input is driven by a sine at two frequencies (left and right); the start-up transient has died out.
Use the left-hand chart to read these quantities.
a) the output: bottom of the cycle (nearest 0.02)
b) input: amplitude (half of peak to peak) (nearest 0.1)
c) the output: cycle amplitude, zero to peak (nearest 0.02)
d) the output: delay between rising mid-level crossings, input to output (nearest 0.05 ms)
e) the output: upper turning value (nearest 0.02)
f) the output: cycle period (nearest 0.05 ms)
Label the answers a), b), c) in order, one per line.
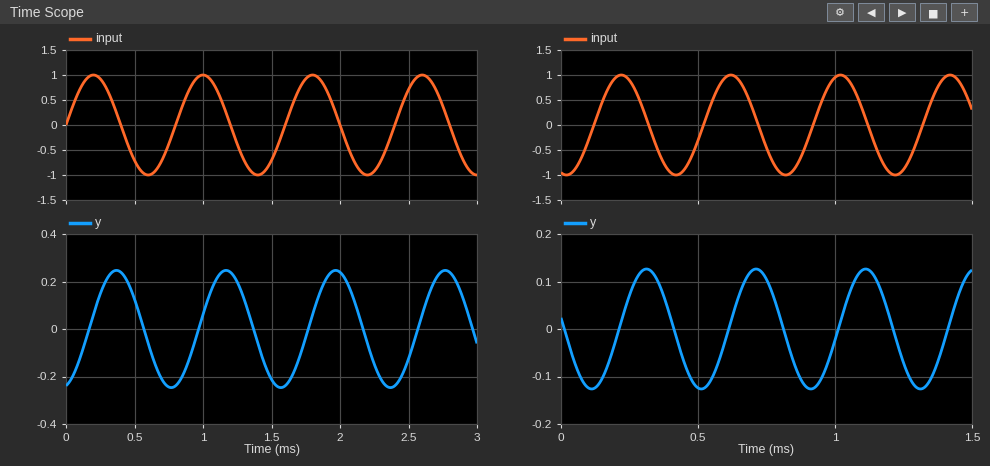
a) -0.24
b) 1.0
c) 0.24
d) 0.15 ms
e) 0.24
f) 0.80 ms
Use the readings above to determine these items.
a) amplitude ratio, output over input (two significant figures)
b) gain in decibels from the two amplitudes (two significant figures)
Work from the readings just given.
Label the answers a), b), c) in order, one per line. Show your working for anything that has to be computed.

a) 0.24 / 1 = 0.24
b) 20 log10(0.24 / 1) = -12 dB
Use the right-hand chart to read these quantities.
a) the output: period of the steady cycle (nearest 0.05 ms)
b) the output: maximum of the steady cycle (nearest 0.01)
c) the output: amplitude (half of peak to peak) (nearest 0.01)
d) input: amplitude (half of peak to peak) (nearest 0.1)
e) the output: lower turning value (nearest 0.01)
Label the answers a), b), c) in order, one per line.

a) 0.40 ms
b) 0.13
c) 0.13
d) 1.0
e) -0.13
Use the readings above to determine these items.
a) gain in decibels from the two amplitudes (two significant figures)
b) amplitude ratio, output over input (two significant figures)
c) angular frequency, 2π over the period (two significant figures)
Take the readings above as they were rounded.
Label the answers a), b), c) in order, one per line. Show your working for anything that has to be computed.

a) 20 log10(0.13 / 1) = -18 dB
b) 0.13 / 1 = 0.13
c) 2π / 0.4 = 16 rad/ms
